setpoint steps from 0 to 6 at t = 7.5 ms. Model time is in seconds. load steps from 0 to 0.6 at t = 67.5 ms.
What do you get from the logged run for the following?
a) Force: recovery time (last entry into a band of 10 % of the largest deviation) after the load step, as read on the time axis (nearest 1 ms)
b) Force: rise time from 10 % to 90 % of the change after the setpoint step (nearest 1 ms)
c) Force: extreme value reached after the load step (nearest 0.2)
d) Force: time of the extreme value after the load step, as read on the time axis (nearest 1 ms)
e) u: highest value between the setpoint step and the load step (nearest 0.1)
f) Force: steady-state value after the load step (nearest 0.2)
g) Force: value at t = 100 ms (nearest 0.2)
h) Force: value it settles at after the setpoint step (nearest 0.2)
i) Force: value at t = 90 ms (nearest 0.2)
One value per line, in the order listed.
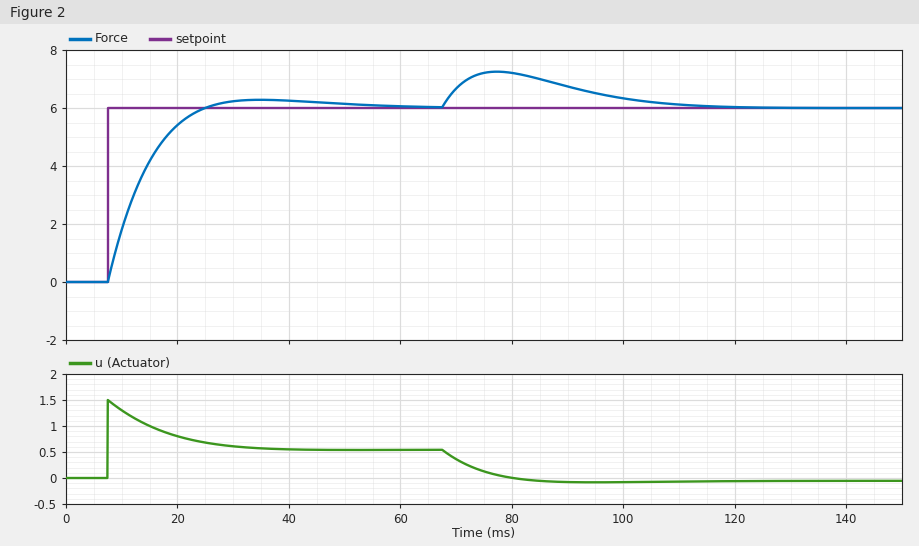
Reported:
110 ms
12 ms
7.2
77 ms
1.5
6.0
6.4
6.0
6.8
